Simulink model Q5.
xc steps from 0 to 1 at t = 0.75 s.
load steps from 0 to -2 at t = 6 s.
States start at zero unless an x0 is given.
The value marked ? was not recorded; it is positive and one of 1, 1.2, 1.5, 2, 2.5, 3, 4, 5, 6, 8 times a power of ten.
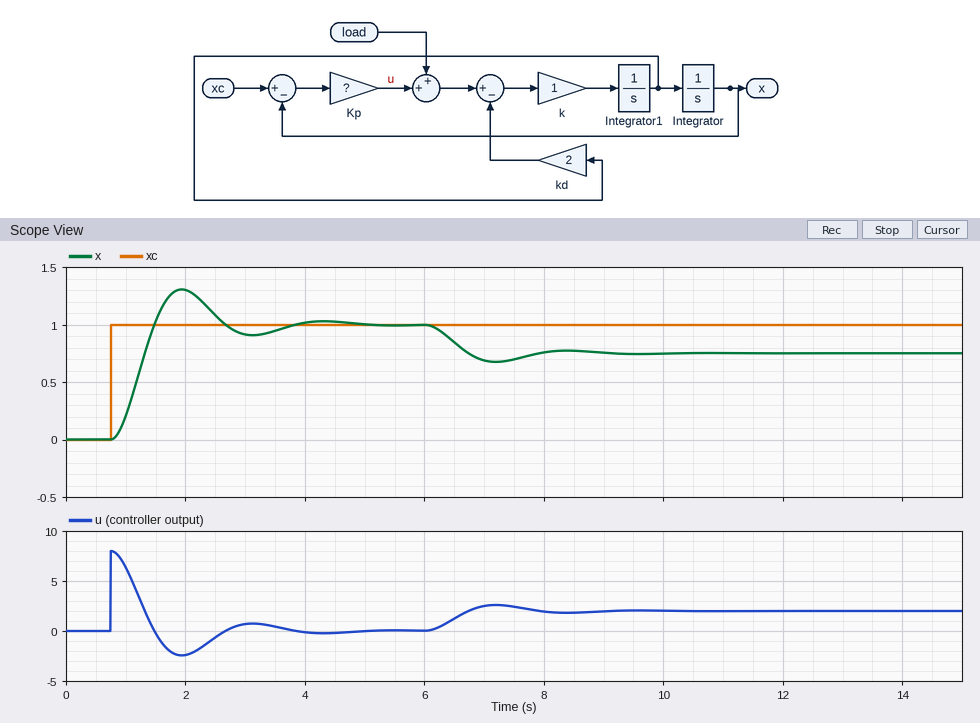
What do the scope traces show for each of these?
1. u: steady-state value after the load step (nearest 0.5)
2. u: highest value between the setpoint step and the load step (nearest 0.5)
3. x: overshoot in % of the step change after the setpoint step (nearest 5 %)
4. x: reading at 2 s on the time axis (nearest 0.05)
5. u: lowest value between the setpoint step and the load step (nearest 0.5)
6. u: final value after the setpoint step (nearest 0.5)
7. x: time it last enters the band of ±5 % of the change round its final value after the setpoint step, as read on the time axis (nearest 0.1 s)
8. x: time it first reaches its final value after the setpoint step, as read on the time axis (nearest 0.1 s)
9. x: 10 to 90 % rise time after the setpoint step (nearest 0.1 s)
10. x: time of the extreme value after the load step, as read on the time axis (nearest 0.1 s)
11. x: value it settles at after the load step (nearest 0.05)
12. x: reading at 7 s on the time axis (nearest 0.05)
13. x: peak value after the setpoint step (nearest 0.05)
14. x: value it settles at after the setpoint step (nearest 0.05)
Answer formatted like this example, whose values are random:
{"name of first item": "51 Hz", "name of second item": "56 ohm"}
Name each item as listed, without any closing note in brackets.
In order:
{"u: steady-state value after the load step": "2.0", "u: highest value between the setpoint step and the load step": "8.0", "x: overshoot in % of the step change after the setpoint step": "30 %", "x: reading at 2 s on the time axis": "1.30", "u: lowest value between the setpoint step and the load step": "-2.5", "u: final value after the setpoint step": "0.0", "x: time it last enters the band of ±5 % of the change round its final value after the setpoint step, as read on the time axis": "3.5 s", "x: time it first reaches its final value after the setpoint step, as read on the time axis": "1.5 s", "x: 10 to 90 % rise time after the setpoint step": "0.5 s", "x: time of the extreme value after the load step, as read on the time axis": "7.2 s", "x: value it settles at after the load step": "0.75", "x: reading at 7 s on the time axis": "0.70", "x: peak value after the setpoint step": "1.30", "x: value it settles at after the setpoint step": "1.00"}
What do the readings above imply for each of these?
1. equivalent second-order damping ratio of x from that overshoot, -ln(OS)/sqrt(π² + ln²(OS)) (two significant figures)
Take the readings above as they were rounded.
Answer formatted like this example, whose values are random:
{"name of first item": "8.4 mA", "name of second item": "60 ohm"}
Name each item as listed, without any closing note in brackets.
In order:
{"equivalent second-order damping ratio of x from that overshoot, -ln(OS)/sqrt(π² + ln²(OS))": "0.36"}
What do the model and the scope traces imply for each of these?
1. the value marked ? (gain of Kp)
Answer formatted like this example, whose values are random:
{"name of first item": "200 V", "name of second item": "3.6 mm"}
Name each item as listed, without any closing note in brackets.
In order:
{"the value marked ?": "8"}
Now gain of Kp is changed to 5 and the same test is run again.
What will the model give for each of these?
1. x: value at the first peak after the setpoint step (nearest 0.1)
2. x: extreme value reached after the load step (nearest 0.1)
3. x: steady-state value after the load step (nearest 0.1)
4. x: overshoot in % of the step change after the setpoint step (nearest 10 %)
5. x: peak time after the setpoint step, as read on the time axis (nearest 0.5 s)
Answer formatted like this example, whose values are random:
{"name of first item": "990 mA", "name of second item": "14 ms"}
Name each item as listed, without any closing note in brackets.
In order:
{"x: value at the first peak after the setpoint step": "1.2", "x: extreme value reached after the load step": "0.5", "x: steady-state value after the load step": "0.6", "x: overshoot in % of the step change after the setpoint step": "20 %", "x: peak time after the setpoint step, as read on the time axis": "2.5 s"}
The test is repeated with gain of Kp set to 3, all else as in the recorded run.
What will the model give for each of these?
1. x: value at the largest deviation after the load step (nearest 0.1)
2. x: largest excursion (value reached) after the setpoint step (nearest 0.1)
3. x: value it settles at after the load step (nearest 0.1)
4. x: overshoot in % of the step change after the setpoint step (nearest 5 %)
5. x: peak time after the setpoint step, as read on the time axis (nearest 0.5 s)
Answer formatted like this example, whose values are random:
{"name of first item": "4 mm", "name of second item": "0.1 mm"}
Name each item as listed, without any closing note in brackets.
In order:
{"x: value at the largest deviation after the load step": "0.3", "x: largest excursion (value reached) after the setpoint step": "1.1", "x: value it settles at after the load step": "0.3", "x: overshoot in % of the step change after the setpoint step": "10 %", "x: peak time after the setpoint step, as read on the time axis": "3.0 s"}
